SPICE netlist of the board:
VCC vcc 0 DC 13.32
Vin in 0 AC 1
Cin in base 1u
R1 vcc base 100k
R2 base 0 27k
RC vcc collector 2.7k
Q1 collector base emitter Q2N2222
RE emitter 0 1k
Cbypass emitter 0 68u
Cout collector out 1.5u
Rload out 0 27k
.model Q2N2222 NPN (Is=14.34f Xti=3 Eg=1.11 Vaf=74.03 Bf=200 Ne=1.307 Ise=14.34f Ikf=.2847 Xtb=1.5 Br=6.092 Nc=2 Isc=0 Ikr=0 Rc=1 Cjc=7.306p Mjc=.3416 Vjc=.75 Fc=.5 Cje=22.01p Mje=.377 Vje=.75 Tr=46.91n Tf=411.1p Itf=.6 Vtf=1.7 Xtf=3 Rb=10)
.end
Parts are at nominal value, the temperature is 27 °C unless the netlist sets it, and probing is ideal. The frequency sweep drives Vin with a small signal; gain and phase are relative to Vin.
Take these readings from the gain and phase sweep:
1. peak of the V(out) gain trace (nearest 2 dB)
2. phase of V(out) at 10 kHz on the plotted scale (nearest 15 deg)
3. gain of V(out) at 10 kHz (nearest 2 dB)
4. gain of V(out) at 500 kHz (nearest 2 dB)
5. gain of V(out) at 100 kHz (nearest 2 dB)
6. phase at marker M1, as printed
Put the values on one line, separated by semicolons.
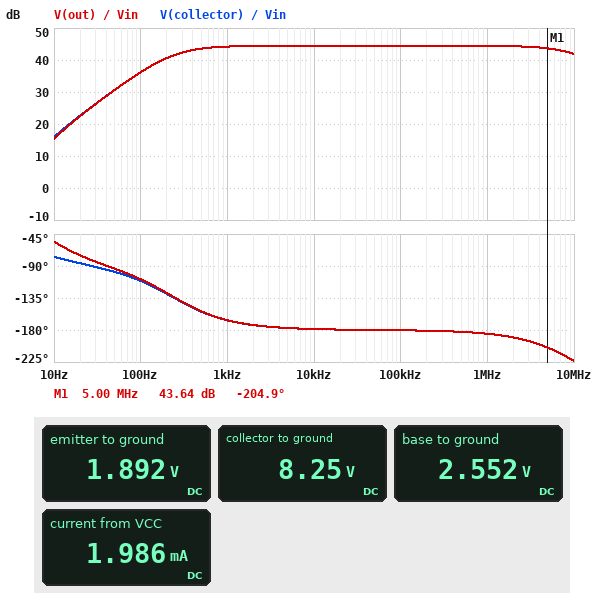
44 dB; -180 deg; 44 dB; 44 dB; 44 dB; -204.9 deg
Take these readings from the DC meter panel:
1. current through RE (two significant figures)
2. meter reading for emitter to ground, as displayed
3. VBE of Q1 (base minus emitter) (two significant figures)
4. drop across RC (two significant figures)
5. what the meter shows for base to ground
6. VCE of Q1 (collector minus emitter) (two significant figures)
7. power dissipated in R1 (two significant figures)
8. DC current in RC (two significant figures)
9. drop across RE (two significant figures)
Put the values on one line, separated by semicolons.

1.9 mA; 1.892 V; 660 mV; 5.1 V; 2.552 V; 6.4 V; 1.2 mW; 1.9 mA; 1.9 V
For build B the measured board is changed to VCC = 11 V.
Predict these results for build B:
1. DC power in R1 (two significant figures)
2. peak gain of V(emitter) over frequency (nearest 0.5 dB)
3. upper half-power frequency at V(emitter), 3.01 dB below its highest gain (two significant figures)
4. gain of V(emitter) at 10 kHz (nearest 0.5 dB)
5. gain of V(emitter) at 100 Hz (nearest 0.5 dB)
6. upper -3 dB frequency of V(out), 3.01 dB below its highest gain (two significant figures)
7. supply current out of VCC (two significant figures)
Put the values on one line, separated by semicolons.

790 µW; -4.0 dB; 200 Hz; -38.0 dB; -4.5 dB; 12 MHz; 1.5 mA
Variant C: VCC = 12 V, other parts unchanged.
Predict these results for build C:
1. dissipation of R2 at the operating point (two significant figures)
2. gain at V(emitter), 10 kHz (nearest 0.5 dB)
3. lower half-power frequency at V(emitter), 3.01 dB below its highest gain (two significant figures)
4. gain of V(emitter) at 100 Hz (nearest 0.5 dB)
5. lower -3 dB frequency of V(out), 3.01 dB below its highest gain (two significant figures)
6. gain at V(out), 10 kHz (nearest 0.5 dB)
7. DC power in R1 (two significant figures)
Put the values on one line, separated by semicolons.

200 µW; -37.0 dB; 5.5 Hz; -4.5 dB; 210 Hz; 43.5 dB; 940 µW
